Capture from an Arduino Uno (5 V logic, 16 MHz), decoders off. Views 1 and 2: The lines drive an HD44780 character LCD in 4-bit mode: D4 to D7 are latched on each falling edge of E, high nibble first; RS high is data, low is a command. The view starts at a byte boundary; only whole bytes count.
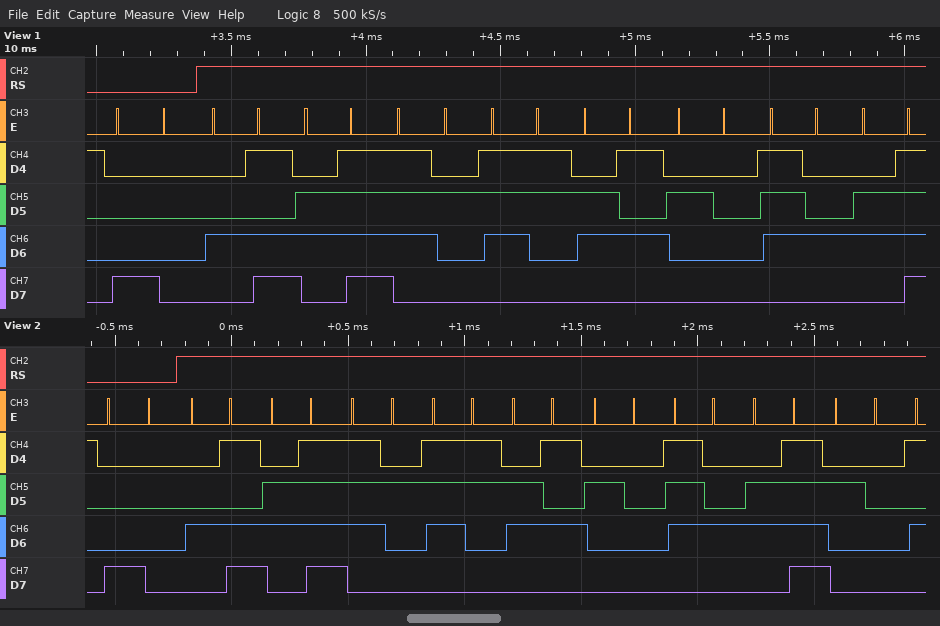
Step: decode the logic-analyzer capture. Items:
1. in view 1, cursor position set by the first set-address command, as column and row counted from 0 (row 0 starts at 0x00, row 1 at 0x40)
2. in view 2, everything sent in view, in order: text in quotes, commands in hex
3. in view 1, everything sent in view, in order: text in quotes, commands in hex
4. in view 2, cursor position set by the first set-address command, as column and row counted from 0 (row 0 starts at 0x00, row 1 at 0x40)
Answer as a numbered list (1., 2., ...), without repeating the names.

1. column 0, row 0
2. 0x80 "Morse to "
3. 0x80 "Morse to"
4. column 0, row 0
